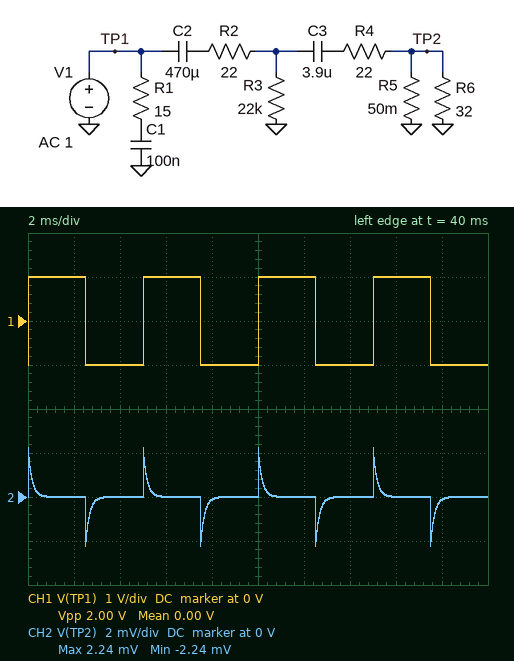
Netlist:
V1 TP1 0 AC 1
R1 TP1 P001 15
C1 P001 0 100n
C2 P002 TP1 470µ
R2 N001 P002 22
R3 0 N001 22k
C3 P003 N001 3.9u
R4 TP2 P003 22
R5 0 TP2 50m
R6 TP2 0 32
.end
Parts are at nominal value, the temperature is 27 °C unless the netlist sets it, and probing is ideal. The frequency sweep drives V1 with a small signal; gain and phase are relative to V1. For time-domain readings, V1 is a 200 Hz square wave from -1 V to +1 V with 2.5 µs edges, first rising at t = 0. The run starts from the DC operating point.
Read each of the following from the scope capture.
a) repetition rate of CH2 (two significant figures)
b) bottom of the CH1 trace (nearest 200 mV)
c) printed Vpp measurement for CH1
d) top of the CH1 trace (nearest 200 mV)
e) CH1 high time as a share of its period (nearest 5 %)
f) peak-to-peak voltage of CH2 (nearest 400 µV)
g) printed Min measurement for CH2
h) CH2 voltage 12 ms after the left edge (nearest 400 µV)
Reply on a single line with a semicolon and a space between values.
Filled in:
200 Hz; -1.0 V; 2.00 V; 1.0 V; 50 %; 4.4 mV; -2.24 mV; 0 V
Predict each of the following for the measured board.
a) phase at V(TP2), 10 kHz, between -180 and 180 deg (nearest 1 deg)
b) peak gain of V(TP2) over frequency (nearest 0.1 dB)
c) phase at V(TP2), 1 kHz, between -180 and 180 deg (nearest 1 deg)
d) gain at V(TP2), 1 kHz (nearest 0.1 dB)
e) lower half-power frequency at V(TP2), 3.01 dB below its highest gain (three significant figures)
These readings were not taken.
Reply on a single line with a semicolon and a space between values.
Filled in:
5 deg; -58.9 dB; 43 deg; -61.6 dB; 935 Hz
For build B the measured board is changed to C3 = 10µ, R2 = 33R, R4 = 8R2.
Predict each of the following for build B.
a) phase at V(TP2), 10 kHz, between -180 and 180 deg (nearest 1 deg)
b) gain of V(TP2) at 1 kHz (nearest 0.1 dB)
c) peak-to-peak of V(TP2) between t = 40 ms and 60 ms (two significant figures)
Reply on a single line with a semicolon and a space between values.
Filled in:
2 deg; -59.0 dB; 4.8 mV
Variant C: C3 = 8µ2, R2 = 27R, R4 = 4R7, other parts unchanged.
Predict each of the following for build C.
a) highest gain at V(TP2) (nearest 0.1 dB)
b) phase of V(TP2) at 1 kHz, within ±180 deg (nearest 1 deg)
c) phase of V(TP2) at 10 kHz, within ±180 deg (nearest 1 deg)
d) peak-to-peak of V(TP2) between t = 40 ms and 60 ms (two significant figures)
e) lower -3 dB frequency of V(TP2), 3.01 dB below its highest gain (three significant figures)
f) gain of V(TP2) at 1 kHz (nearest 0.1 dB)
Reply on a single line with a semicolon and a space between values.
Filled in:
-56.1 dB; 32 deg; 4 deg; 6.3 mV; 623 Hz; -57.5 dB
